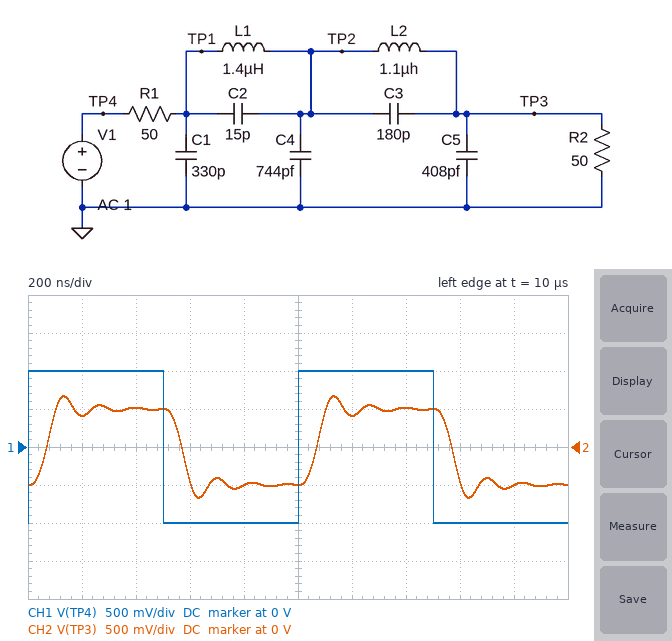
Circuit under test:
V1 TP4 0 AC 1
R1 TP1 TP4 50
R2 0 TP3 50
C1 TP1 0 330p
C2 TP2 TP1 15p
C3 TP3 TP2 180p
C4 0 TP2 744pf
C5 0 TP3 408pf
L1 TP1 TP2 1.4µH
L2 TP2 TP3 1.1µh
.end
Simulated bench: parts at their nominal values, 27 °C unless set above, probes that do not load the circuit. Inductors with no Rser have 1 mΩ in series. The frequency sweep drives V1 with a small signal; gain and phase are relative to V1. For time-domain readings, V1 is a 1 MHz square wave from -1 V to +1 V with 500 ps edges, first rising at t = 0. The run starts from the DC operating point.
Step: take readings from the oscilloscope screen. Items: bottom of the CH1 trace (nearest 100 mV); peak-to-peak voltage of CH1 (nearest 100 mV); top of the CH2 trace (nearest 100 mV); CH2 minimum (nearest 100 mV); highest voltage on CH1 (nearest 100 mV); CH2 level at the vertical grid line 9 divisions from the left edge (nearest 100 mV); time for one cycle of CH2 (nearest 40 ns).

-1.0 V
2.0 V
700 mV
-700 mV
1.0 V
-500 mV
1.00 µs
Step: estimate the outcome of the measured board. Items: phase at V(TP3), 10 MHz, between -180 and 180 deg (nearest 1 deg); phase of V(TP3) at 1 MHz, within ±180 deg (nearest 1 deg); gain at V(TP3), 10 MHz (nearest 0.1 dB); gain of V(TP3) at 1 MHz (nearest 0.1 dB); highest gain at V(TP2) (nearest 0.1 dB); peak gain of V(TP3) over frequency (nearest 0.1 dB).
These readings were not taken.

23 deg
-22 deg
-30.1 dB
-6.0 dB
-1.4 dB
-6.0 dB
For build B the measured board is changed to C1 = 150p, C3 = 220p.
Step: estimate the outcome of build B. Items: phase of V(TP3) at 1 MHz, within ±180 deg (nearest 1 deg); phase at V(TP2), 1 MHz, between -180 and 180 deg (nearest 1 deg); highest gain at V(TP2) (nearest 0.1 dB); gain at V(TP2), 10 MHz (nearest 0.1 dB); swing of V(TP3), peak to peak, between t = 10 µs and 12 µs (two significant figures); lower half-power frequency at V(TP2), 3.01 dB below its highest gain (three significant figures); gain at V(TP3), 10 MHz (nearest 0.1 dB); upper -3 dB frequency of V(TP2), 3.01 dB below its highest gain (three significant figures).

-21 deg
-13 deg
-2.0 dB
-10.9 dB
1.3 V
5.63 MHz
-44.8 dB
8.23 MHz
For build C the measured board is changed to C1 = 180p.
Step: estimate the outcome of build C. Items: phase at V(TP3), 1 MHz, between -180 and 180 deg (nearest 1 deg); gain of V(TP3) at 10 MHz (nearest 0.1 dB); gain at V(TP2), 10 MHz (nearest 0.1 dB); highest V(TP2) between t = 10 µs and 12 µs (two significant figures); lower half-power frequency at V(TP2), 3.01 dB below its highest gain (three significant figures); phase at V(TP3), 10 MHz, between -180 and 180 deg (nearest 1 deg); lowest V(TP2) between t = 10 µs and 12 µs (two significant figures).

-21 deg
-29.6 dB
-10.1 dB
650 mV
5.80 MHz
49 deg
-650 mV
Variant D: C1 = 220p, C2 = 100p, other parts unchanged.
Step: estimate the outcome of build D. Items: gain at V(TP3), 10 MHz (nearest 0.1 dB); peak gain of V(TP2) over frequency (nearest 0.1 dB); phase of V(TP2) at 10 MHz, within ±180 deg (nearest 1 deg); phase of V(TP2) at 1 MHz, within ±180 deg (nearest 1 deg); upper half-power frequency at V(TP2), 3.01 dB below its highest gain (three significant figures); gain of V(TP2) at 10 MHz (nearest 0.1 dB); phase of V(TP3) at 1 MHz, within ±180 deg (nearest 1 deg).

-37.8 dB
-2.7 dB
158 deg
-13 deg
7.93 MHz
-18.2 dB
-21 deg
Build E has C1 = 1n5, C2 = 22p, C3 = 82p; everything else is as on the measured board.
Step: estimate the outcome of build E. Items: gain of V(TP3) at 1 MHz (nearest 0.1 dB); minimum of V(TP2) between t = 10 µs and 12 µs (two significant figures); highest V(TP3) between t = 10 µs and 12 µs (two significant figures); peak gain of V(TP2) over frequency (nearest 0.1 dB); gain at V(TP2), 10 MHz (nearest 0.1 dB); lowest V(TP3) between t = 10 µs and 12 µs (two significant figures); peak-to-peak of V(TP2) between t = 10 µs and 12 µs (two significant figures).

-6.3 dB
-520 mV
550 mV
-6.0 dB
-20.5 dB
-550 mV
1.0 V
